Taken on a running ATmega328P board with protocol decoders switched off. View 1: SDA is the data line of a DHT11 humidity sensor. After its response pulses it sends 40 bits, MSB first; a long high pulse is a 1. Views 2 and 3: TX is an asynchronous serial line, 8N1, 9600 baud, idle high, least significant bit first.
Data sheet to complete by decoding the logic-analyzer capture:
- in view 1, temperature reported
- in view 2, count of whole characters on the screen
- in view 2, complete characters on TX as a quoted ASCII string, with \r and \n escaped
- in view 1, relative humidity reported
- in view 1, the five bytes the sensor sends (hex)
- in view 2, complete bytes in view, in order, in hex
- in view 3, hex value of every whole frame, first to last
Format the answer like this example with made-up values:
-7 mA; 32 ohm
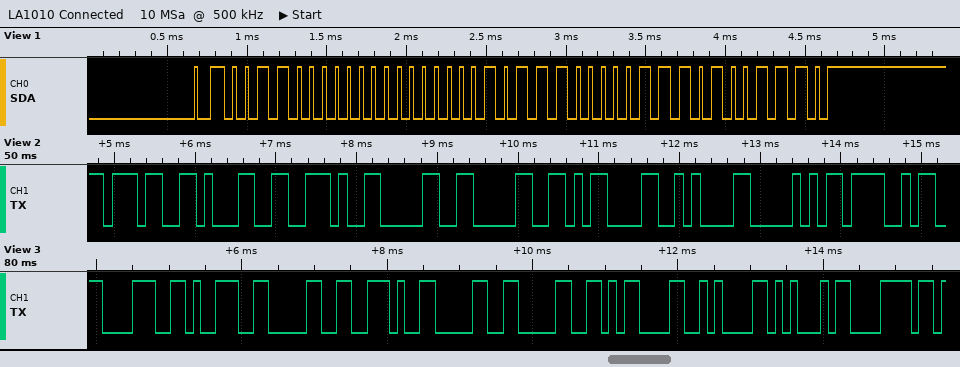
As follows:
23.7 °C; 9; "71.00\r\nPO"; 48 %; 30 00 17 07 4E; 37 31 2E 30 30 0D 0A 50 4F; 38 39 30 2E 30 30 0D 0A 45 78
